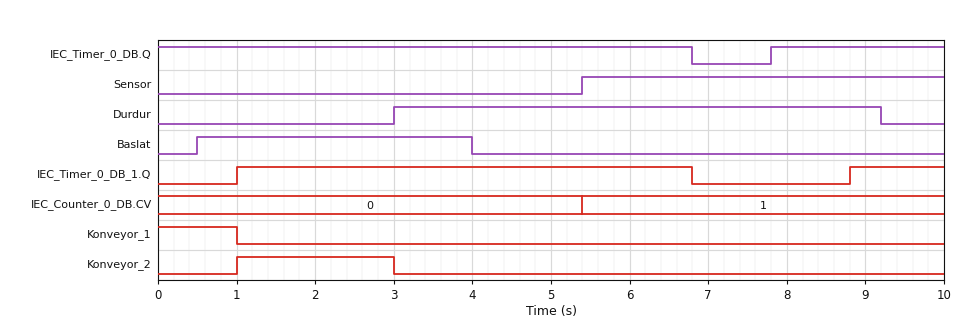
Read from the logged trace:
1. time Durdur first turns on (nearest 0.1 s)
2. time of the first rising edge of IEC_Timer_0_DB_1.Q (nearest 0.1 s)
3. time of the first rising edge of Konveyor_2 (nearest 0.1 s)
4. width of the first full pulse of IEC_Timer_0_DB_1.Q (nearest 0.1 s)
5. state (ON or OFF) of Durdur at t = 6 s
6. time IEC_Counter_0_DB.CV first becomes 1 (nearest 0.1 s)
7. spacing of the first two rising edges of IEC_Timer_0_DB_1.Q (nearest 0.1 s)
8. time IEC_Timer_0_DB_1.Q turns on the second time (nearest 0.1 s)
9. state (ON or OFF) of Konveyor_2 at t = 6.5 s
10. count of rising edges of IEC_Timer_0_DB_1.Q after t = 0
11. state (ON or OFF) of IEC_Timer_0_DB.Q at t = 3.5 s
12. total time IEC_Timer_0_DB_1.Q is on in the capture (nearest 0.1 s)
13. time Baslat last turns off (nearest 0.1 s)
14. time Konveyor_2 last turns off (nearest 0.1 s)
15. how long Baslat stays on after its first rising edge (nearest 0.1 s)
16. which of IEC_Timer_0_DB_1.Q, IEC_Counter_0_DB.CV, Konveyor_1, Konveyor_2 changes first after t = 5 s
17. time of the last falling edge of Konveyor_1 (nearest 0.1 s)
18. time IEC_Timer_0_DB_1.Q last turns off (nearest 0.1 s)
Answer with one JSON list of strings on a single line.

["3.0 s", "1.0 s", "1.0 s", "5.8 s", "ON", "5.4 s", "7.8 s", "8.8 s", "OFF", "2", "ON", "7.0 s", "4.0 s", "3.0 s", "3.5 s", "IEC_Counter_0_DB.CV", "1.0 s", "6.8 s"]
